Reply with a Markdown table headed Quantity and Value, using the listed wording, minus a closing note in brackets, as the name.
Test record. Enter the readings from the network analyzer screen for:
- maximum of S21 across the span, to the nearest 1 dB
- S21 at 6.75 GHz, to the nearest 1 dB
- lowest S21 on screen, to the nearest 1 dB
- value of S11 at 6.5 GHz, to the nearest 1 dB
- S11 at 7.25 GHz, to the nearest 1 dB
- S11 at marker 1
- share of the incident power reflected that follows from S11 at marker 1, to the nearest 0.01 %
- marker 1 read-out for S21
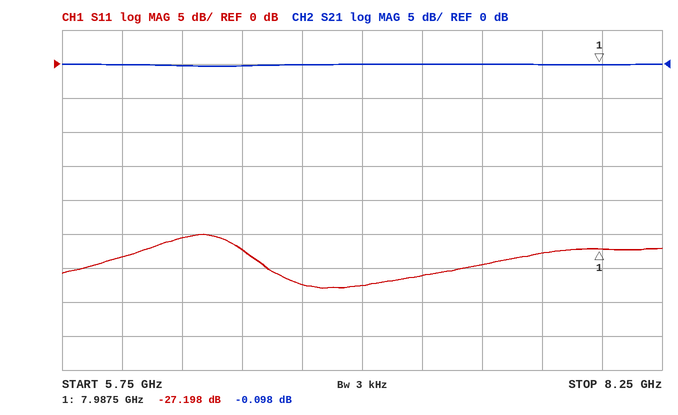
| Quantity | Value |
|---|---|
| maximum of S21 across the span, to the nearest 1 dB | 0 dB |
| S21 at 6.75 GHz, to the nearest 1 dB | 0 dB |
| lowest S21 on screen, to the nearest 1 dB | 0 dB |
| value of S11 at 6.5 GHz, to the nearest 1 dB | -27 dB |
| S11 at 7.25 GHz, to the nearest 1 dB | -31 dB |
| S11 at marker 1 | -27.198 dB |
| share of the incident power reflected that follows from S11 at marker 1, to the nearest 0.01 % | 0.19 % |
| marker 1 read-out for S21 | -0.098 dB |
